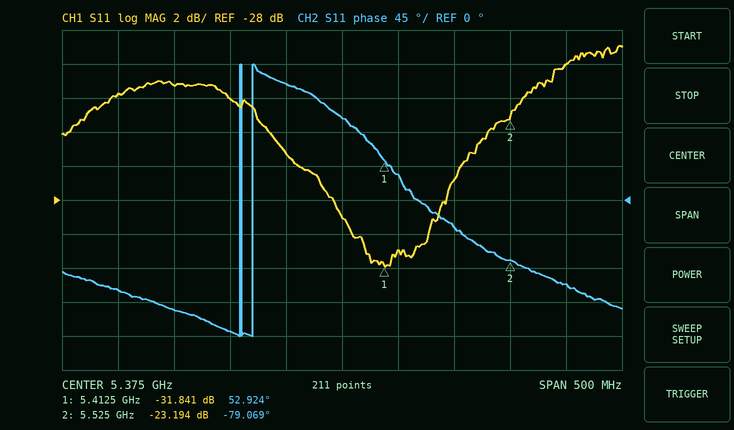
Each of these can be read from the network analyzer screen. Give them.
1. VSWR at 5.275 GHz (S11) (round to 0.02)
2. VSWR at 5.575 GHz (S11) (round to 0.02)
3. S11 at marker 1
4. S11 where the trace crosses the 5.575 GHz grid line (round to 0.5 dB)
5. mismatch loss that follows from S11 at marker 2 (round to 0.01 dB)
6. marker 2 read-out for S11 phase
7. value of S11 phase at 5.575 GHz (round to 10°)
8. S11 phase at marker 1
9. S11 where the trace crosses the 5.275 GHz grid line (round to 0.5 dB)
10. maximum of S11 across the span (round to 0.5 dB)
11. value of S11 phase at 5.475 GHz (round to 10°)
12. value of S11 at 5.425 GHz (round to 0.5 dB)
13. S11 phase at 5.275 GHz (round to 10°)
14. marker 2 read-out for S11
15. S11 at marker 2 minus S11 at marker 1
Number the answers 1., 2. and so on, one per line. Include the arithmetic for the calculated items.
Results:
1. |Γ| = 10^(-22/20) = 0.0794; VSWR = (1 + 0.0794)/(1 − 0.0794) ≈ 1.17, so 1.18 to the nearest 0.02
2. |Γ| = 10^(-20/20) = 0.1000; VSWR = (1 + 0.1000)/(1 − 0.1000) ≈ 1.22
3. -31.841 dB
4. -20.0 dB
5. −10 log10(1 − 10^(-23.194/10)) ≈ 0.02 dB
6. -79.069°
7. -110°
8. 52.924°
9. -22.0 dB
10. -19.0 dB
11. -40°
12. -31.0 dB
13. -170°
14. -23.194 dB
15. -23.194 − (-31.841) = 8.647 dB
